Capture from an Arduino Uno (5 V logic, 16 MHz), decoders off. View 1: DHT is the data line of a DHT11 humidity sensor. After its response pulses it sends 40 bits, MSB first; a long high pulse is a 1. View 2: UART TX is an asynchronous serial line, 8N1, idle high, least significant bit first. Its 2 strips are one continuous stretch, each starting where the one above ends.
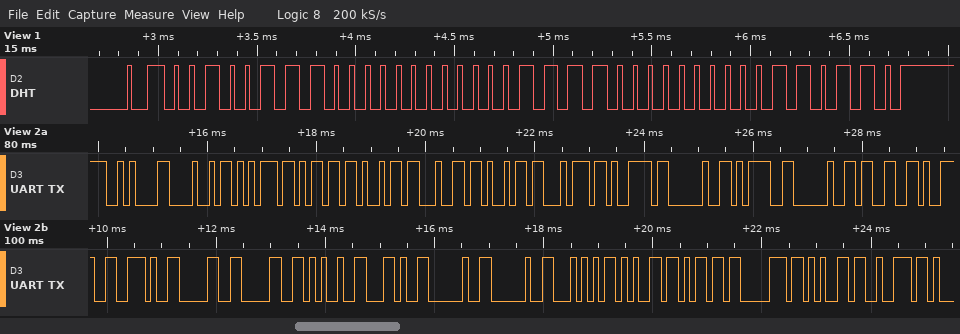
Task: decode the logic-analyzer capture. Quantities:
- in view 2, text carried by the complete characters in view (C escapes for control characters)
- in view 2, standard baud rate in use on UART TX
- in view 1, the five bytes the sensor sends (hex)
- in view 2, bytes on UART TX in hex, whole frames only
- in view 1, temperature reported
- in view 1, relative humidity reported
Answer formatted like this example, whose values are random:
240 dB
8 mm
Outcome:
"\nHumidity = 39.00%,  Temper"
9600 baud
27 00 0F 00 36
0A 48 75 6D 69 64 69 74 79 20 3D 20 33 39 2E 30 30 25 2C 20 20 54 65 6D 70 65 72
15.0 °C
39 %
